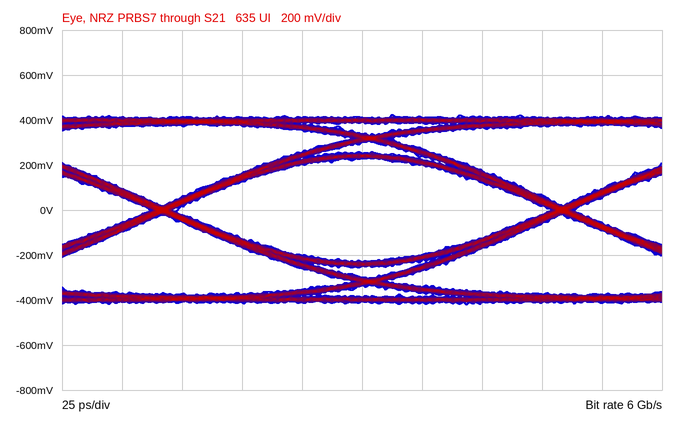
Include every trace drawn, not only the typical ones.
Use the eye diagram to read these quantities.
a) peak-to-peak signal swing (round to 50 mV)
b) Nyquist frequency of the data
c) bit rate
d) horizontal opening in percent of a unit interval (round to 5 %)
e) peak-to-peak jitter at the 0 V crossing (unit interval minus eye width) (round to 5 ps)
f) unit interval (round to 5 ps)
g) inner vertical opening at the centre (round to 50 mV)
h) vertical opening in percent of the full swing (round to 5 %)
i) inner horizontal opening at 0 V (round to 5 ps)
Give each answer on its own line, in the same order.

850 mV
3 GHz
6 Gb/s
95 %
10 ps
165 ps
450 mV
55 %
155 ps
